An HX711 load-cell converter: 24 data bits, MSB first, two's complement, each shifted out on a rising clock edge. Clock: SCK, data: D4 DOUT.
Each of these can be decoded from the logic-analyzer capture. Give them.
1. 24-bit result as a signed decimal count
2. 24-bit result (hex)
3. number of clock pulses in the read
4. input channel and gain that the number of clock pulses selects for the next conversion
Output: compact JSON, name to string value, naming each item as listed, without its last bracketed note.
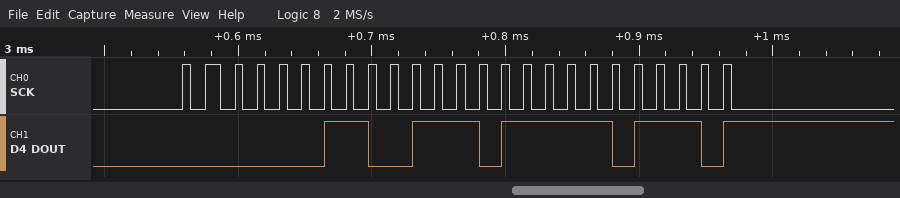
{"24-bit result as a signed decimal count": "211950", "24-bit result": "0x033BEE", "number of clock pulses in the read": "25", "input channel and gain that the number of clock pulses selects for the next conversion": "channel A, gain 128"}
